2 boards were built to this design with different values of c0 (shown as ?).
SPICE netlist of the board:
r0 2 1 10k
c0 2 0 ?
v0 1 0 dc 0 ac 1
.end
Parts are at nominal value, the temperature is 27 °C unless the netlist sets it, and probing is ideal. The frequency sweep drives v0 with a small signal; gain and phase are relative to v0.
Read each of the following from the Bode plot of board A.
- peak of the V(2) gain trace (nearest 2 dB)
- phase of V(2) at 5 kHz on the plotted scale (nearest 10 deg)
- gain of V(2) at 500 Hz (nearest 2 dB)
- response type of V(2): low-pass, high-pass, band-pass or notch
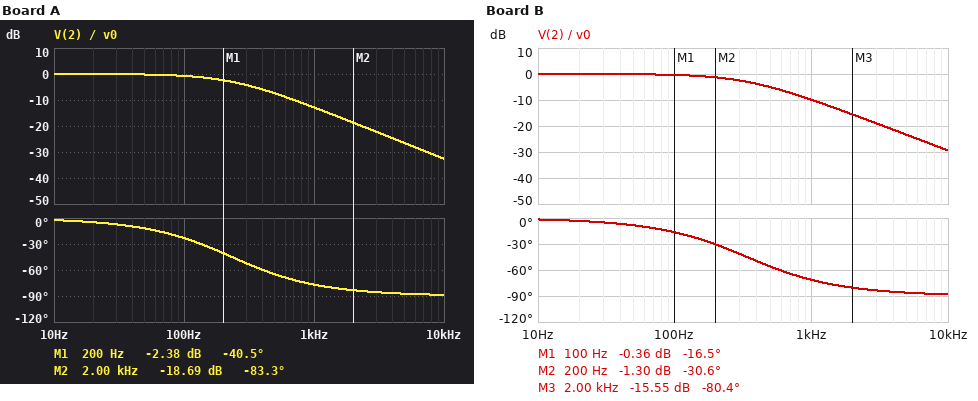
0 dB
-90 deg
-8 dB
low-pass
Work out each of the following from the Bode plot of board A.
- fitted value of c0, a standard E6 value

68 nF
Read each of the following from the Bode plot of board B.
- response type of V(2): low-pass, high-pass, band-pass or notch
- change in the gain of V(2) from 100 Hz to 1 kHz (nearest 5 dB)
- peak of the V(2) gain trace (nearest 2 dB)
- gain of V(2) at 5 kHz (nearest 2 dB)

low-pass
-10 dB
0 dB
-24 dB
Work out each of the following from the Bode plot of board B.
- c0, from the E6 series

47 nF
